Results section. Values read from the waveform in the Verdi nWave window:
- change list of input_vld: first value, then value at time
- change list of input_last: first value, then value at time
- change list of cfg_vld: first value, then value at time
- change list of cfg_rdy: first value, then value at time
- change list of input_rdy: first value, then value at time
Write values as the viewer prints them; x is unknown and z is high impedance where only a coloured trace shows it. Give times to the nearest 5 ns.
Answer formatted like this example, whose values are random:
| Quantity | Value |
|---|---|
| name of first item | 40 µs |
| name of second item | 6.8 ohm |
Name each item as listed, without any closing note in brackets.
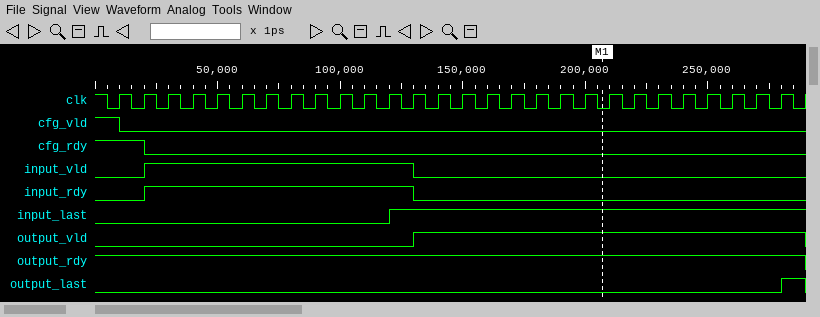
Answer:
| Quantity | Value |
|---|---|
| change list of input_vld: first value, then value at time | 0, 1 at 20 ns, 0 at 130 ns |
| change list of input_last: first value, then value at time | 0, 1 at 120 ns |
| change list of cfg_vld: first value, then value at time | 1, 0 at 10 ns |
| change list of cfg_rdy: first value, then value at time | 1, 0 at 20 ns |
| change list of input_rdy: first value, then value at time | 0, 1 at 20 ns, 0 at 130 ns |
